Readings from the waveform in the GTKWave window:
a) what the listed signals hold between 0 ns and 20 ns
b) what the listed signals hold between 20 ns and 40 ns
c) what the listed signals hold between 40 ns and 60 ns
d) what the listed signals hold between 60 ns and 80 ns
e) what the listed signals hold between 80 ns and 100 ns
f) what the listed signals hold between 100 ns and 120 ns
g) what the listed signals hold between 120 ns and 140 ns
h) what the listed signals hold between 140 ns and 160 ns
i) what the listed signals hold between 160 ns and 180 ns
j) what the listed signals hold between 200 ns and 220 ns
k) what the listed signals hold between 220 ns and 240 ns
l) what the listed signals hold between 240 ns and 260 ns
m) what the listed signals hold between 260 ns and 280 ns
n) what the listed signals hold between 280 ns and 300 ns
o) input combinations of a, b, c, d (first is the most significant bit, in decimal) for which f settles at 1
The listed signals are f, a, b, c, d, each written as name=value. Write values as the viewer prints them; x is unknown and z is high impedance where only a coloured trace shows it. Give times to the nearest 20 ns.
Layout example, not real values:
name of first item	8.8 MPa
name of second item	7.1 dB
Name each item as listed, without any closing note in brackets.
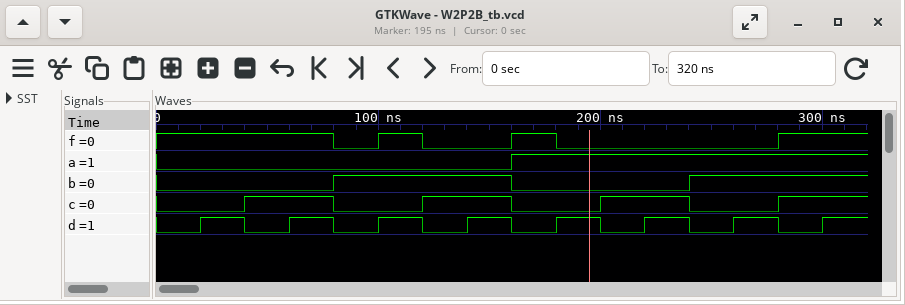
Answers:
what the listed signals hold between 0 ns and 20 ns	f=1, a=0, b=0, c=0, d=0
what the listed signals hold between 20 ns and 40 ns	f=1, a=0, b=0, c=0, d=1
what the listed signals hold between 40 ns and 60 ns	f=1, a=0, b=0, c=1, d=0
what the listed signals hold between 60 ns and 80 ns	f=1, a=0, b=0, c=1, d=1
what the listed signals hold between 80 ns and 100 ns	f=0, a=0, b=1, c=0, d=0
what the listed signals hold between 100 ns and 120 ns	f=1, a=0, b=1, c=0, d=1
what the listed signals hold between 120 ns and 140 ns	f=0, a=0, b=1, c=1, d=0
what the listed signals hold between 140 ns and 160 ns	f=0, a=0, b=1, c=1, d=1
what the listed signals hold between 160 ns and 180 ns	f=1, a=1, b=0, c=0, d=0
what the listed signals hold between 200 ns and 220 ns	f=0, a=1, b=0, c=1, d=0
what the listed signals hold between 220 ns and 240 ns	f=0, a=1, b=0, c=1, d=1
what the listed signals hold between 240 ns and 260 ns	f=0, a=1, b=1, c=0, d=0
what the listed signals hold between 260 ns and 280 ns	f=0, a=1, b=1, c=0, d=1
what the listed signals hold between 280 ns and 300 ns	f=1, a=1, b=1, c=1, d=0
input combinations of a, b, c, d (first is the most significant bit, in decimal) for which f settles at 1	0, 1, 2, 3, 5, 8, 14, 15
